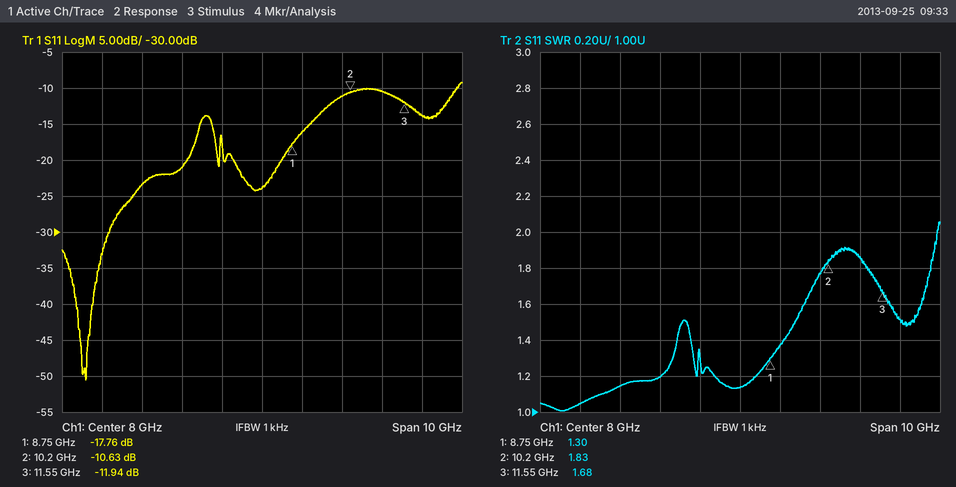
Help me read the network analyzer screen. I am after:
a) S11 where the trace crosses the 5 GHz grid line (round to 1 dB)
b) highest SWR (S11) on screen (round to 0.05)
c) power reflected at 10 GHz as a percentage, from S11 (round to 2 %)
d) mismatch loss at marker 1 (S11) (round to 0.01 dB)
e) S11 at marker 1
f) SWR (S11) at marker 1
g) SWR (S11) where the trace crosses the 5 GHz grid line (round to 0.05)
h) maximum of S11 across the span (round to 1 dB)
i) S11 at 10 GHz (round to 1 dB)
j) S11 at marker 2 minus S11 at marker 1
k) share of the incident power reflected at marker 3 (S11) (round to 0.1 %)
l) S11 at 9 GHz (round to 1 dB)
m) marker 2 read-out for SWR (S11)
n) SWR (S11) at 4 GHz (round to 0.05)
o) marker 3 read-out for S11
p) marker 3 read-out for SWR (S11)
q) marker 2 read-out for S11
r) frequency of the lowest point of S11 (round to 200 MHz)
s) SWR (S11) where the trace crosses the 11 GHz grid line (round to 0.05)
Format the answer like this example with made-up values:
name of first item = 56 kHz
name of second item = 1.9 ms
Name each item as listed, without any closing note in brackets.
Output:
S11 where the trace crosses the 5 GHz grid line = -23 dB
highest SWR (S11) on screen = 2.05
power reflected at 10 GHz as a percentage, from S11 = 8 %
mismatch loss at marker 1 (S11) = 0.07 dB
S11 at marker 1 = -17.76 dB
SWR (S11) at marker 1 = 1.30
SWR (S11) where the trace crosses the 5 GHz grid line = 1.15
maximum of S11 across the span = -9 dB
S11 at 10 GHz = -11 dB
S11 at marker 2 minus S11 at marker 1 = 7.13 dB
share of the incident power reflected at marker 3 (S11) = 6.4 %
S11 at 9 GHz = -16 dB
marker 2 read-out for SWR = 1.83
SWR (S11) at 4 GHz = 1.05
marker 3 read-out for S11 = -11.94 dB
marker 3 read-out for SWR = 1.68
marker 2 read-out for S11 = -10.63 dB
frequency of the lowest point of S11 = 3.6 GHz
SWR (S11) where the trace crosses the 11 GHz grid line = 1.85
